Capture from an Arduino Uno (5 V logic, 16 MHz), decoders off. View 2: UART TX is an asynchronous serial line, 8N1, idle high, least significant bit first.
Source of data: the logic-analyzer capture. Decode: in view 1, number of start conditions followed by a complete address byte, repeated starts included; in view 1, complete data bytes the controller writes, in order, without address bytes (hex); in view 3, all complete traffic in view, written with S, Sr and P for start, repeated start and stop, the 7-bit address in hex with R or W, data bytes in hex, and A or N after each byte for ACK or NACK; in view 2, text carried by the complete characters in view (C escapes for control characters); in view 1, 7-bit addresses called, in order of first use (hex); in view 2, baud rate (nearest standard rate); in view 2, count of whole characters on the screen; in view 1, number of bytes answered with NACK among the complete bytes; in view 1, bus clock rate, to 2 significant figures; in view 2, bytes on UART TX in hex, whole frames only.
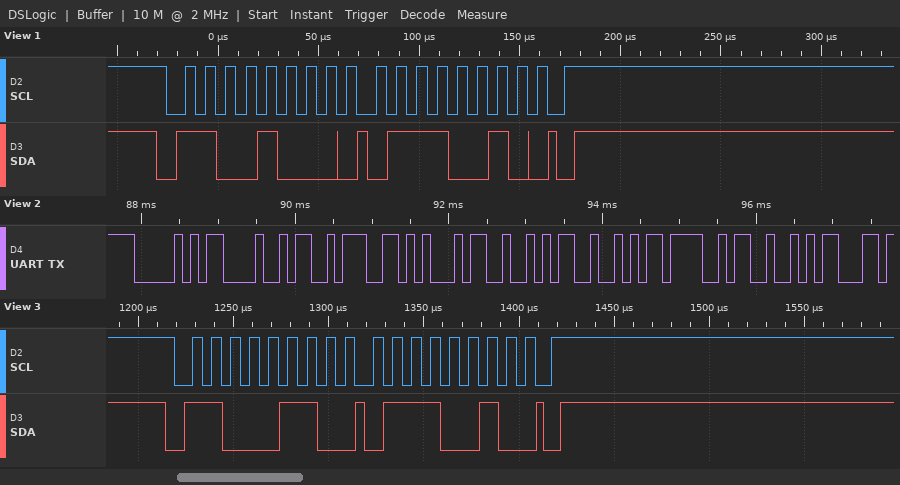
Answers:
1
72
S 63W A 72 A P
"PH:ERROR"
0x64
9600 baud
8
0
100 kHz
50 48 3A 45 52 52 4F 52
